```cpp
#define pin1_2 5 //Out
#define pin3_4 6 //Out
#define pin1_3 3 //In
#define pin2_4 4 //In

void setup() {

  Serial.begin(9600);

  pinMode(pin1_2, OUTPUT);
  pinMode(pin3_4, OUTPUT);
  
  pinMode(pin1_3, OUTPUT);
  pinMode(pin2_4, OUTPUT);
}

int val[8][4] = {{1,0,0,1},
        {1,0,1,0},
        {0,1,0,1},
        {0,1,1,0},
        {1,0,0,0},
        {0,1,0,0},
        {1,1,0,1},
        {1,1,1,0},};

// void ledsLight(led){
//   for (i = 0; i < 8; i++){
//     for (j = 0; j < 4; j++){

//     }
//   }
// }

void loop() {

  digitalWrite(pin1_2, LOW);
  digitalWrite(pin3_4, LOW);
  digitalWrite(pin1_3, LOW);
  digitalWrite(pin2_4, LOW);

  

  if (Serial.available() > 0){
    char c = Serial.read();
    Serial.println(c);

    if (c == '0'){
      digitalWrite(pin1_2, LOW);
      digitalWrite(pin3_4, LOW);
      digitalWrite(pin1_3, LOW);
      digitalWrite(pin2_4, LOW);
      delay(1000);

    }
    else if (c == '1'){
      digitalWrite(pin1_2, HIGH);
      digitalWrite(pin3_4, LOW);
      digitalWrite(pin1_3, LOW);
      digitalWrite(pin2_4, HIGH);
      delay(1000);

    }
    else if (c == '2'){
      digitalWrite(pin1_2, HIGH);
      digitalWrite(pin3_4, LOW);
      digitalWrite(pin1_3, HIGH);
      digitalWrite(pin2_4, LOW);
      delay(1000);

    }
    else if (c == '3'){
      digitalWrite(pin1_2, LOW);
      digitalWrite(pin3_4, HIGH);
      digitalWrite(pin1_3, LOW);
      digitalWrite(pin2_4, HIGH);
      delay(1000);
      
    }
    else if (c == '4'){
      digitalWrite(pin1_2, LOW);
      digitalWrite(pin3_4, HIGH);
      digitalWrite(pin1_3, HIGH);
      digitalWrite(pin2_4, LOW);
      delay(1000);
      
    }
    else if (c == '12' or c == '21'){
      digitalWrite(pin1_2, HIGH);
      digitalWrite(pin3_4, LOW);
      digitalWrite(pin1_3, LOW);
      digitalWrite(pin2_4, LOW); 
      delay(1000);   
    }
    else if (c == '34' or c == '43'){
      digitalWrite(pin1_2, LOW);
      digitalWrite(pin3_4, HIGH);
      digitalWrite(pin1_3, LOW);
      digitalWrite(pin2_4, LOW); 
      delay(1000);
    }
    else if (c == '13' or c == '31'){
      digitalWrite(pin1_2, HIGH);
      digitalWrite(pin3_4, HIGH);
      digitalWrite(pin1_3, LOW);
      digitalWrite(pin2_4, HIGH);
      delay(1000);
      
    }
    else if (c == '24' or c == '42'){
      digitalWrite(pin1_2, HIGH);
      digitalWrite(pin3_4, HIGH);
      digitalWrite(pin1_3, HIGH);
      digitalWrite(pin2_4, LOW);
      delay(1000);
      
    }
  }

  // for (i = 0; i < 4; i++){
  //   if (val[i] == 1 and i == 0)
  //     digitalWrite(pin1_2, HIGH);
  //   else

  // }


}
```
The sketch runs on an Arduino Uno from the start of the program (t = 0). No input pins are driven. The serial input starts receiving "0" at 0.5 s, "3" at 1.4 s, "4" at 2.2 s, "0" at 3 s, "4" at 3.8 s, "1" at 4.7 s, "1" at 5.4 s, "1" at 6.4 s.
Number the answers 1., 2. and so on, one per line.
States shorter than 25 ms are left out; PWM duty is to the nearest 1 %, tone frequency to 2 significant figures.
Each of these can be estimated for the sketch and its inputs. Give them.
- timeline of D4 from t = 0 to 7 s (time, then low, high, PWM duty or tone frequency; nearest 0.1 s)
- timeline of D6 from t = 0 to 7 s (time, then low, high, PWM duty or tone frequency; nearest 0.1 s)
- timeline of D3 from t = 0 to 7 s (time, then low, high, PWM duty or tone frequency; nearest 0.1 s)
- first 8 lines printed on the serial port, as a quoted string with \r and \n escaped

1. 0 s low; 1.5 s high; 2.5 s low; 5.5 s high
2. 0 s low; 1.5 s high; 3.5 s low; 4.5 s high; 5.5 s low
3. 0 s low; 2.5 s high; 3.5 s low; 4.5 s high; 5.5 s low
4. "0\r\n3\r\n4\r\n0\r\n4\r\n1\r\n1\r\n1\r\n"
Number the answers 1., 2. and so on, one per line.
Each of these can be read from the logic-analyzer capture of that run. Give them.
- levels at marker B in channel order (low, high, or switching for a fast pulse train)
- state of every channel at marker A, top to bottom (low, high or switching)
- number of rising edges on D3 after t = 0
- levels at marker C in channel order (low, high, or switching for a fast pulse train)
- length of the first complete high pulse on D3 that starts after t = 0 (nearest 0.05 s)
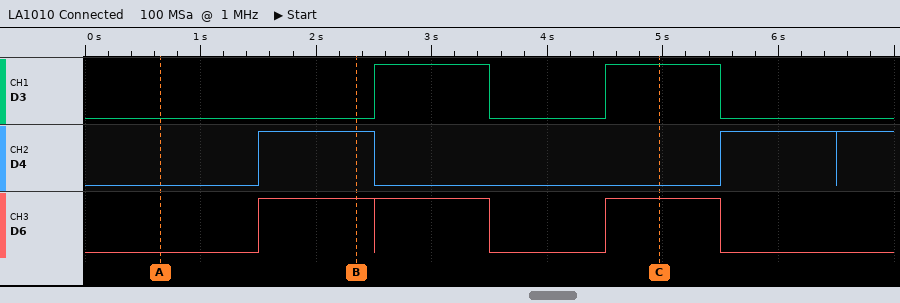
1. D3 low, D4 high, D6 high
2. D3 low, D4 low, D6 low
3. 2
4. D3 high, D4 low, D6 high
5. 1.00 s
